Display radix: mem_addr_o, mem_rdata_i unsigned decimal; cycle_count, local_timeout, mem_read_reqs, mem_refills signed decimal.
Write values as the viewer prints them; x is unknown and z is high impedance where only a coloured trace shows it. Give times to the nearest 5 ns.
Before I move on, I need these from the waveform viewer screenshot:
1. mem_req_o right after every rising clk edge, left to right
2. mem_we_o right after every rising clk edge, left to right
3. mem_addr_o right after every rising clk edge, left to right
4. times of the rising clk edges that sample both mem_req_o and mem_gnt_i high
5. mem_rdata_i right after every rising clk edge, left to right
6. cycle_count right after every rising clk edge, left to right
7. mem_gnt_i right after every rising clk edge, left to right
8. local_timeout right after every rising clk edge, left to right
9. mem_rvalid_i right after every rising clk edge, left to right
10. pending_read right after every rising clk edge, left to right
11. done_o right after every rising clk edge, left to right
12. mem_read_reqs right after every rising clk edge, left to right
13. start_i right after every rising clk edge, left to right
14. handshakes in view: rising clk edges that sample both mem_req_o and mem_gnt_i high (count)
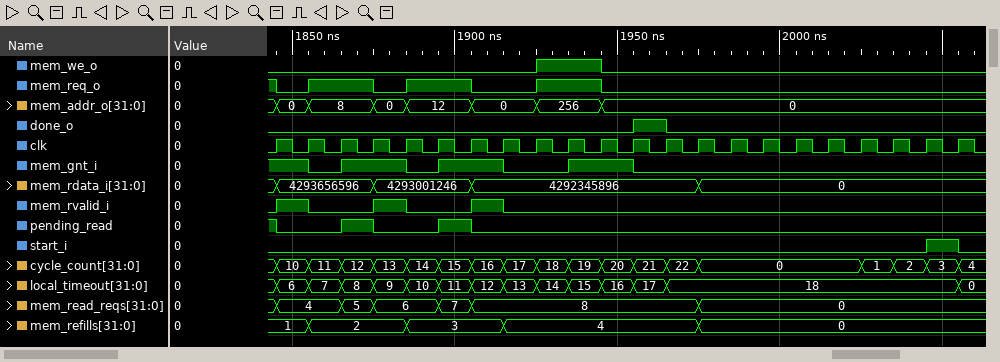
0 1 1 0 1 1 0 0 1 1 0 0 0 0 0 0 0 0 0 0 0 0
0 0 0 0 0 0 0 0 1 1 0 0 0 0 0 0 0 0 0 0 0 0
0, 8, 8, 0, 12, 12, 0, 0, 256, 256, 0, 0, 0, 0, 0, 0, 0, 0, 0, 0, 0, 0
1845 ns, 1875 ns, 1905 ns, 1945 ns
4293656596, 4293656596, 4293656596, 4293001246, 4293001246, 4293001246, 4292345896, 4292345896, 4292345896, 4292345896, 4292345896, 4292345896, 4292345896, 0, 0, 0, 0, 0, 0, 0, 0, 0
10, 11, 12, 13, 14, 15, 16, 17, 18, 19, 20, 21, 22, 0, 0, 0, 0, 0, 1, 2, 3, 4
1 0 1 1 0 1 1 0 0 1 1 0 0 0 0 0 0 0 0 0 0 0
6, 7, 8, 9, 10, 11, 12, 13, 14, 15, 16, 17, 18, 18, 18, 18, 18, 18, 18, 18, 18, 0
1 0 0 1 0 0 1 0 0 0 0 0 0 0 0 0 0 0 0 0 0 0
0 0 1 0 0 1 0 0 0 0 0 0 0 0 0 0 0 0 0 0 0 0
0 0 0 0 0 0 0 0 0 0 0 1 0 0 0 0 0 0 0 0 0 0
4, 4, 5, 6, 6, 7, 8, 8, 8, 8, 8, 8, 8, 0, 0, 0, 0, 0, 0, 0, 0, 0
0 0 0 0 0 0 0 0 0 0 0 0 0 0 0 0 0 0 0 0 1 0
4
